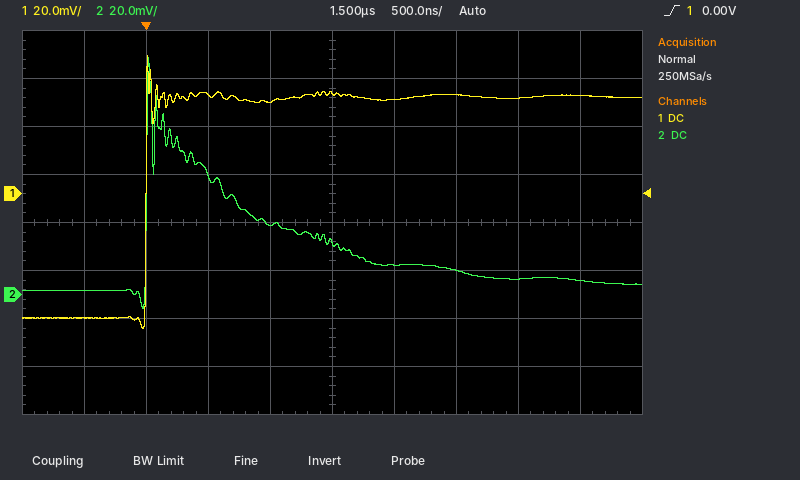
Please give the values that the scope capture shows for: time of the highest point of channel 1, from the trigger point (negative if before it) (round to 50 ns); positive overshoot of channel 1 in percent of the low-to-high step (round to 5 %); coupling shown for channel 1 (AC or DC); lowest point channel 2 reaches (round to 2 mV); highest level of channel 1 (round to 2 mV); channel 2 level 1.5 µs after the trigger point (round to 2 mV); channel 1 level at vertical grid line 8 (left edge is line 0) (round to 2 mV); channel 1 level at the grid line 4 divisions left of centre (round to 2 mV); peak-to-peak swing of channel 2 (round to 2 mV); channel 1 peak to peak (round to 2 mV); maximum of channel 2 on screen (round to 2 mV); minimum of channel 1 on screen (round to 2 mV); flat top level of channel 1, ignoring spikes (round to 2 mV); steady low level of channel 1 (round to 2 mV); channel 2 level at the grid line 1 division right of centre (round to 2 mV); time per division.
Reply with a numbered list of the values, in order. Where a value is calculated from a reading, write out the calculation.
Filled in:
1. 0 ns
2. 20 %
3. DC
4. -6 mV
5. 58 mV
6. 22 mV
7. 40 mV
8. -52 mV
9. 98 mV − (-6 mV) = 104 mV
10. 58 mV − (-56 mV) = 114 mV
11. 98 mV
12. -56 mV
13. 40 mV
14. -52 mV
15. 12 mV
16. 500 ns
